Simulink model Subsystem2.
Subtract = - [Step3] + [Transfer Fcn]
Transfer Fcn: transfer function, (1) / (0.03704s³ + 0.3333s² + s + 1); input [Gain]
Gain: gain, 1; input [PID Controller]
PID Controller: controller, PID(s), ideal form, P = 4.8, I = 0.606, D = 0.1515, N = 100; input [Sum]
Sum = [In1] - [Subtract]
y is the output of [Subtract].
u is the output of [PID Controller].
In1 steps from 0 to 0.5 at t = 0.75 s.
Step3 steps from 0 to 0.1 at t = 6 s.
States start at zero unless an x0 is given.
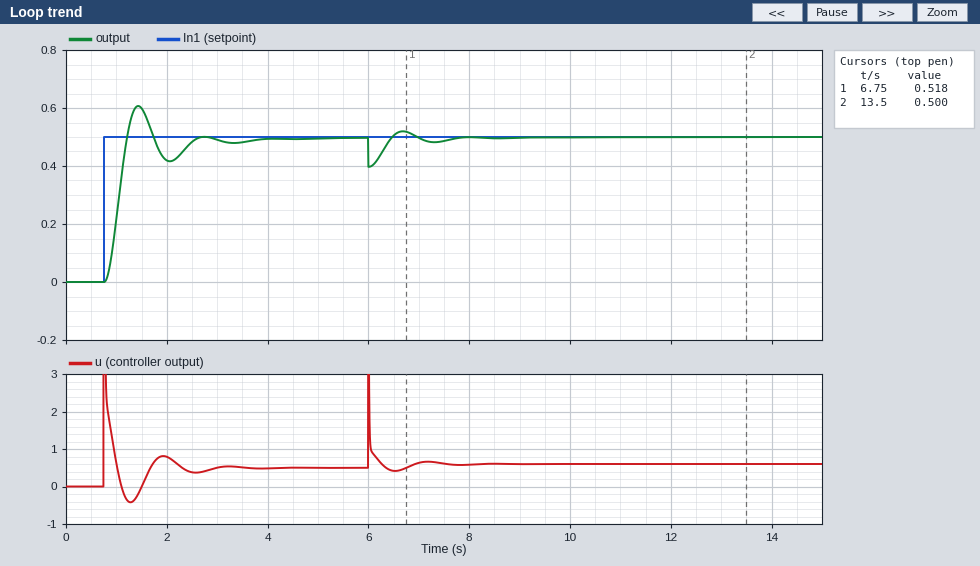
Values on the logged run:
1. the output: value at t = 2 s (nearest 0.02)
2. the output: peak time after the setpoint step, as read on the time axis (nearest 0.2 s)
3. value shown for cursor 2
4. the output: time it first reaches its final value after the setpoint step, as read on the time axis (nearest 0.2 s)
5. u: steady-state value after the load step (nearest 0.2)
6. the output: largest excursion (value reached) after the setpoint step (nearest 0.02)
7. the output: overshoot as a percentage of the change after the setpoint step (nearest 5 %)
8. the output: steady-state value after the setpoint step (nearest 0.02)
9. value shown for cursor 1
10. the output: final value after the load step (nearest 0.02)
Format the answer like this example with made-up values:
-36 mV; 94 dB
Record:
0.42; 1.4 s; 0.500; 1.2 s; 0.6; 0.60; 20 %; 0.50; 0.518; 0.50
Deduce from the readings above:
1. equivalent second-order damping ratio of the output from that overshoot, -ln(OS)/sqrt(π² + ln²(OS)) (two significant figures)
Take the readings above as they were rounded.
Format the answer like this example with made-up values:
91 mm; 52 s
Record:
0.46
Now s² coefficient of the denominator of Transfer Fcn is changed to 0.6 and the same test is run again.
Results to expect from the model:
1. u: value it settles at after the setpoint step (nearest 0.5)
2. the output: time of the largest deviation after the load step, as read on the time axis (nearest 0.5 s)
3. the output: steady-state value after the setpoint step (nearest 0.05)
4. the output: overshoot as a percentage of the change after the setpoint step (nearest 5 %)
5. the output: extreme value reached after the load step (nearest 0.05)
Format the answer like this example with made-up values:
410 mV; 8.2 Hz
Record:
0.5; 6.0 s; 0.50; 25 %; 0.40
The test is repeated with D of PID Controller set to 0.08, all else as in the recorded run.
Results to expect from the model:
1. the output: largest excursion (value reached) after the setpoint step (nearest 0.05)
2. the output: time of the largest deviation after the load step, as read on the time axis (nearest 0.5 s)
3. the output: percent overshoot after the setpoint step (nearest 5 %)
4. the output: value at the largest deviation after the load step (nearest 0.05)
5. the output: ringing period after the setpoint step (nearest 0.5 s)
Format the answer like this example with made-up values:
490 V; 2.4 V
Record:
0.65; 6.0 s; 35 %; 0.40; 1.5 s
